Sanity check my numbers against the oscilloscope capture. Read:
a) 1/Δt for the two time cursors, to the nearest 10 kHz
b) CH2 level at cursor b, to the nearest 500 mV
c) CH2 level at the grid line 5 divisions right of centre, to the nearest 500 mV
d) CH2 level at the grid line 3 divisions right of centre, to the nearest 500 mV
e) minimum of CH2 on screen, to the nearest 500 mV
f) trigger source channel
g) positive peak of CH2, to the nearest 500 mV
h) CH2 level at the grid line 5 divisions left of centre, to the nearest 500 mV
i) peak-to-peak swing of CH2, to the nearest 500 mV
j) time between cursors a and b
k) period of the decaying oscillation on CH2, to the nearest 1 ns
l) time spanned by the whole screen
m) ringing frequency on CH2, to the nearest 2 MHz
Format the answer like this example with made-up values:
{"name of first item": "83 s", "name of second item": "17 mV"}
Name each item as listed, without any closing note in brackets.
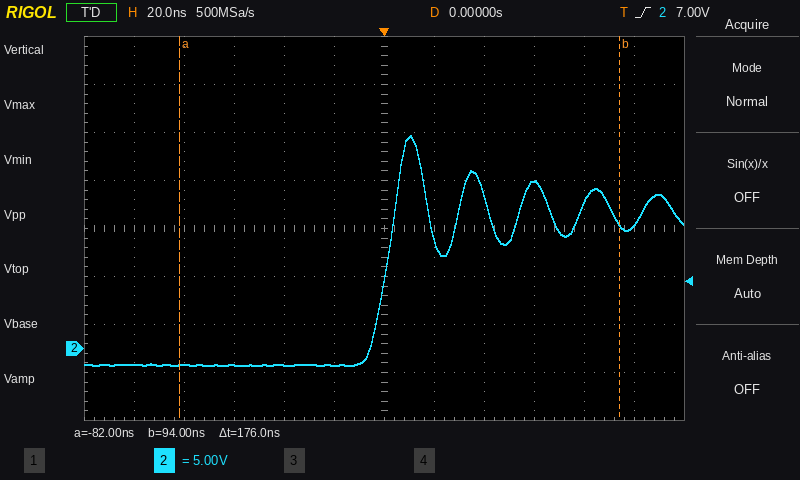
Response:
{"1/Δt for the two time cursors, to the nearest 10 kHz": "5.68 MHz", "CH2 level at cursor b, to the nearest 500 mV": "13.0 V", "CH2 level at the grid line 5 divisions right of centre, to the nearest 500 mV": "13.0 V", "CH2 level at the grid line 3 divisions right of centre, to the nearest 500 mV": "17.5 V", "minimum of CH2 on screen, to the nearest 500 mV": "-2.0 V", "trigger source channel": "CH2", "positive peak of CH2, to the nearest 500 mV": "22.0 V", "CH2 level at the grid line 5 divisions left of centre, to the nearest 500 mV": "-1.5 V", "peak-to-peak swing of CH2, to the nearest 500 mV": "24.0 V", "time between cursors a and b": "176 ns", "period of the decaying oscillation on CH2, to the nearest 1 ns": "25 ns", "time spanned by the whole screen": "240 ns", "ringing frequency on CH2, to the nearest 2 MHz": "40 MHz"}
